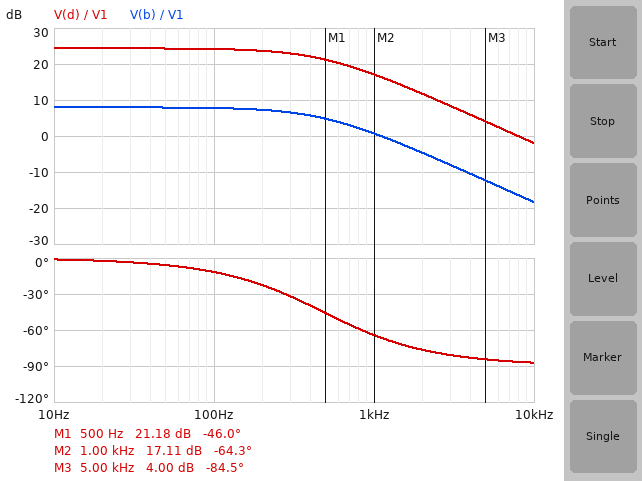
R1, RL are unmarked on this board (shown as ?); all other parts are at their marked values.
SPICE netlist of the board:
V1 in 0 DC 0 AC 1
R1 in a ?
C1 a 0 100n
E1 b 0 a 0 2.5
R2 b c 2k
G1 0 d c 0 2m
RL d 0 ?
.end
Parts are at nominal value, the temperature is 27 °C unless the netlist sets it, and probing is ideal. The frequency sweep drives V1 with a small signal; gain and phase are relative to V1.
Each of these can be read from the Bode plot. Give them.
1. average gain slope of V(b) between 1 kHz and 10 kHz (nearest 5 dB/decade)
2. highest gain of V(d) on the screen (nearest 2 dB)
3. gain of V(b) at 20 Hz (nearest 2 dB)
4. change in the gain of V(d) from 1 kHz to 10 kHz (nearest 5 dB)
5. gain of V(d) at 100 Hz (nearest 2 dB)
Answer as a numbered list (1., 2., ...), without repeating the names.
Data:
1. -20 dB/decade
2. 24 dB
3. 8 dB
4. -20 dB
5. 24 dB
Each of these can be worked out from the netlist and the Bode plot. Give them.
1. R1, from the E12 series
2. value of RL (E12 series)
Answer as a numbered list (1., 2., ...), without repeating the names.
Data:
1. 3.3 kΩ
2. 3.3 kΩ
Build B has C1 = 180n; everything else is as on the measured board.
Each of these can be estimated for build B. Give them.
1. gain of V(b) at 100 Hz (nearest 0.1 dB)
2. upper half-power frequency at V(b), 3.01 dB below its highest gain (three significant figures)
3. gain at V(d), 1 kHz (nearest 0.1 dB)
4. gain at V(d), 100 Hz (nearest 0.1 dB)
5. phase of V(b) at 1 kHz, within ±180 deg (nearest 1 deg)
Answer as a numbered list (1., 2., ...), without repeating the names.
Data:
1. 7.4 dB
2. 268 Hz
3. 12.6 dB
4. 23.8 dB
5. -75 deg
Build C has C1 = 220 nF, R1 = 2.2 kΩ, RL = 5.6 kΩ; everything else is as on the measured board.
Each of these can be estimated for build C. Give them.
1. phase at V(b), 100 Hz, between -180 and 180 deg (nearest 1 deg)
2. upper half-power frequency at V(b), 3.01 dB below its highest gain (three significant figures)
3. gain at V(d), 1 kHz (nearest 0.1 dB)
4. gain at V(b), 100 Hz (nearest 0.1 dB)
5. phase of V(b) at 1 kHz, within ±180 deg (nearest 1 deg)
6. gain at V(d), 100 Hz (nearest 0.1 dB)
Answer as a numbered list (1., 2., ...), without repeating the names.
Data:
1. -17 deg
2. 329 Hz
3. 18.8 dB
4. 7.6 dB
5. -72 deg
6. 28.6 dB
